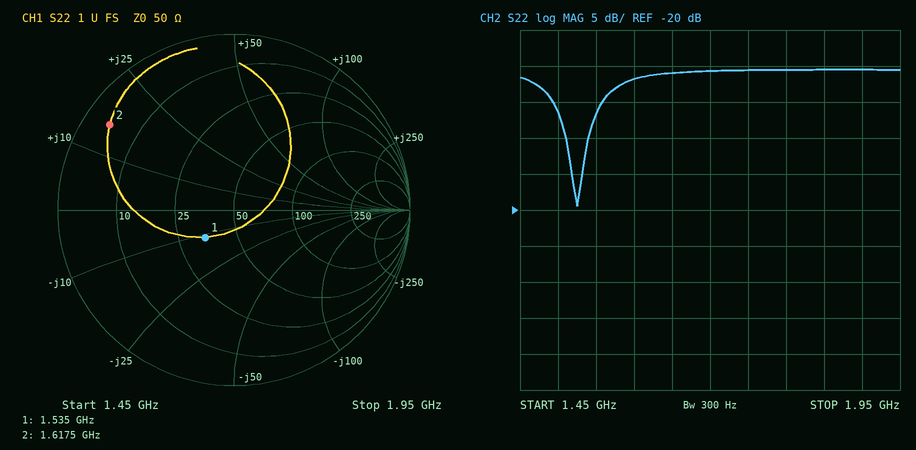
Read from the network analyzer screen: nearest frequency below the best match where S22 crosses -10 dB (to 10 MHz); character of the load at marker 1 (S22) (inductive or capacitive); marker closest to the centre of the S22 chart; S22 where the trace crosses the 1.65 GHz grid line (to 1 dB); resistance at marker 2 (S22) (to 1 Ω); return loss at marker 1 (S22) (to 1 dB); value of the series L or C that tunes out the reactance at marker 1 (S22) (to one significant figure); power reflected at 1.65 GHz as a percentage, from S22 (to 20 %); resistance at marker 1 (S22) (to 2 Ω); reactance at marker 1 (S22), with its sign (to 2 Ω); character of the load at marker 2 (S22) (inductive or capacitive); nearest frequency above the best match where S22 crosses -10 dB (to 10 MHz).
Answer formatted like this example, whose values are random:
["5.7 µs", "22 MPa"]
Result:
["1.51 GHz", "capacitive", "marker 1", "-1 dB", "4 Ω", "13 dB", "1 nH", "80 %", "34 Ω", "-12 Ω", "inductive", "1.54 GHz"]
